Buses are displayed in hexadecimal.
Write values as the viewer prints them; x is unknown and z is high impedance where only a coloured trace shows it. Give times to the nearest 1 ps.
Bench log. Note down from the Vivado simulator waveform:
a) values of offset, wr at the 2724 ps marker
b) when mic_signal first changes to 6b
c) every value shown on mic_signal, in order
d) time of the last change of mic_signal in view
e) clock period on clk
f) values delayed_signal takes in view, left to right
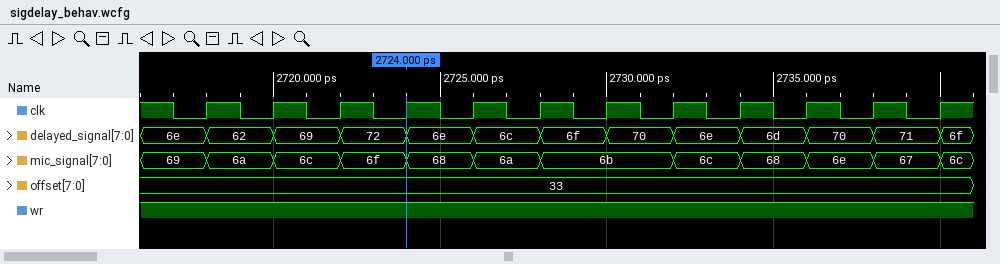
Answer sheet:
offset=33, wr=1
2728 ps
69, 6a, 6c, 6f, 68, 6a, 6b, 6c, 68, 6e, 67, 6c
2740 ps
2 ps
6e, 62, 69, 72, 6e, 6c, 6f, 70, 6e, 6d, 70, 71, 6f
